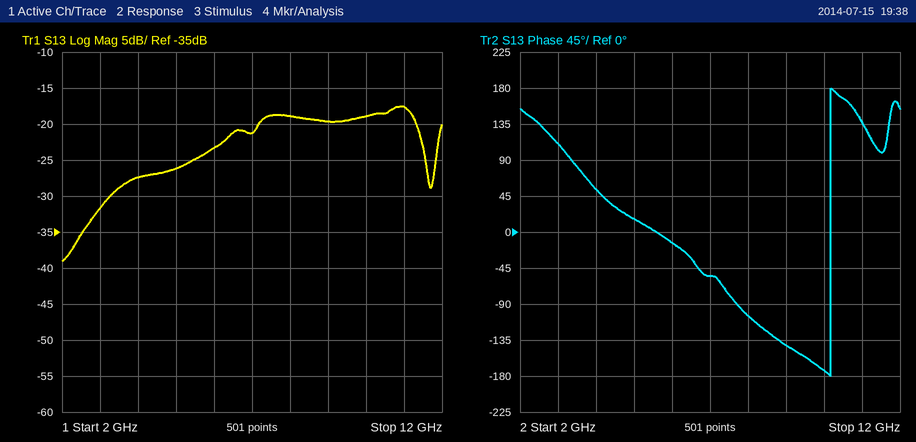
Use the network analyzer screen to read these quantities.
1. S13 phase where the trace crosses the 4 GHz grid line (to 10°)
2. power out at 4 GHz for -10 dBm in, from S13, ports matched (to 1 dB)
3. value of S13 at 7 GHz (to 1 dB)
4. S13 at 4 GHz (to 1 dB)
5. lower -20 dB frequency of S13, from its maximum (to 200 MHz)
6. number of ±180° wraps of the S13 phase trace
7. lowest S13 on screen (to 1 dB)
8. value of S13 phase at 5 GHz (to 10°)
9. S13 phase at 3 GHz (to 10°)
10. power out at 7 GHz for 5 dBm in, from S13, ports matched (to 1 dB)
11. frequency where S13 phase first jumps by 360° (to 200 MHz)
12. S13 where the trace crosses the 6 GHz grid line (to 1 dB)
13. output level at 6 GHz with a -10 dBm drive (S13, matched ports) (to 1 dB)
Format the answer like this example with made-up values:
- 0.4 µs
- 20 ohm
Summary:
- 50°
- -37 dBm
- -21 dB
- -27 dB
- 2.2 GHz
- 1
- -39 dB
- 20°
- 110°
- -16 dBm
- 10.2 GHz
- -23 dB
- -33 dBm
